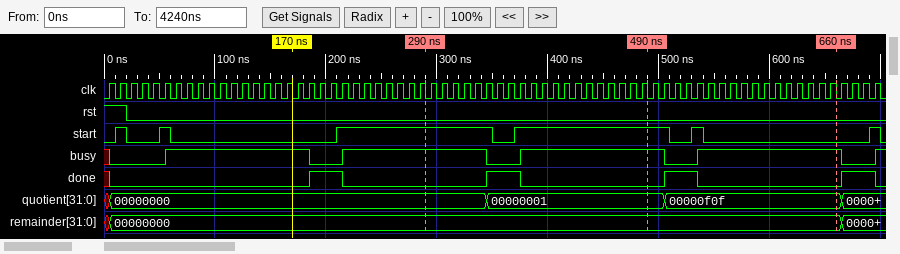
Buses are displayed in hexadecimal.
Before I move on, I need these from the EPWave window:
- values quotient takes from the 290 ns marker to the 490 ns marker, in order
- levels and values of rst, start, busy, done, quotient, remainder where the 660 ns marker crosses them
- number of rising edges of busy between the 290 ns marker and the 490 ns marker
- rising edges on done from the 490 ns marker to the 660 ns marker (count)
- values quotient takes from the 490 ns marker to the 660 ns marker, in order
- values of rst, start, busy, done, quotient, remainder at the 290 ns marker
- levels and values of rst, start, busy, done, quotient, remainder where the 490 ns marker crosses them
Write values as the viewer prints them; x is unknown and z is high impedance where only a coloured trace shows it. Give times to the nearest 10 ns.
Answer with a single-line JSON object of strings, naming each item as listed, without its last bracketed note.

{"values quotient takes from the 290 ns marker to the 490 ns marker, in order": "00000000, 00000001", "levels and values of rst, start, busy, done, quotient, remainder where the 660 ns marker crosses them": "rst=0, start=0, busy=1, done=0, quotient=00000f0f, remainder=00000000", "number of rising edges of busy between the 290 ns marker and the 490 ns marker": "1", "rising edges on done from the 490 ns marker to the 660 ns marker": "1", "values quotient takes from the 490 ns marker to the 660 ns marker, in order": "00000001, 00000f0f", "values of rst, start, busy, done, quotient, remainder at the 290 ns marker": "rst=0, start=1, busy=1, done=0, quotient=00000000, remainder=00000000", "levels and values of rst, start, busy, done, quotient, remainder where the 490 ns marker crosses them": "rst=0, start=1, busy=1, done=0, quotient=00000001, remainder=00000000"}
